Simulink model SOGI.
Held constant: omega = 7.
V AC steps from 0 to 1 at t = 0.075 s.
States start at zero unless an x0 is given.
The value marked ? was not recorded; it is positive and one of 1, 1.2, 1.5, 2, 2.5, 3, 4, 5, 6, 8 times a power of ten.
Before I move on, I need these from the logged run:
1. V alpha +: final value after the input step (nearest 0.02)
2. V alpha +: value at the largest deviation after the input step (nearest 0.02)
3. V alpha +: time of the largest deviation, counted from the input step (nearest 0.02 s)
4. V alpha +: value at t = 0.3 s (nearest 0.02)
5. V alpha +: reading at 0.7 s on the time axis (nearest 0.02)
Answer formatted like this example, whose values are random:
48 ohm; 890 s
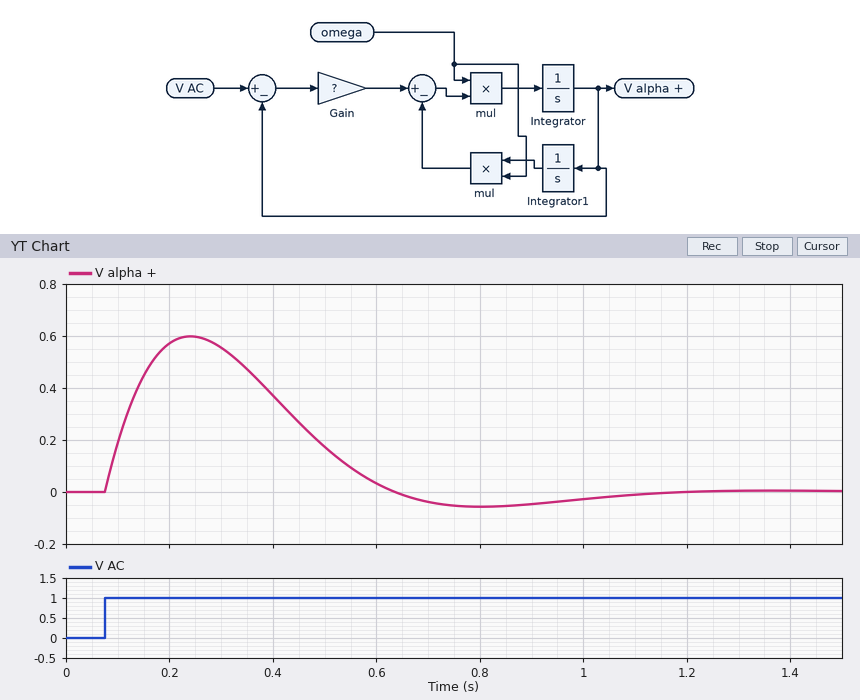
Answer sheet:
0.00; 0.60; 0.16 s; 0.56; -0.04
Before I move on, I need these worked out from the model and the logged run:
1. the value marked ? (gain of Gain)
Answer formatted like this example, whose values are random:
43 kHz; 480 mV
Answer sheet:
1.2
